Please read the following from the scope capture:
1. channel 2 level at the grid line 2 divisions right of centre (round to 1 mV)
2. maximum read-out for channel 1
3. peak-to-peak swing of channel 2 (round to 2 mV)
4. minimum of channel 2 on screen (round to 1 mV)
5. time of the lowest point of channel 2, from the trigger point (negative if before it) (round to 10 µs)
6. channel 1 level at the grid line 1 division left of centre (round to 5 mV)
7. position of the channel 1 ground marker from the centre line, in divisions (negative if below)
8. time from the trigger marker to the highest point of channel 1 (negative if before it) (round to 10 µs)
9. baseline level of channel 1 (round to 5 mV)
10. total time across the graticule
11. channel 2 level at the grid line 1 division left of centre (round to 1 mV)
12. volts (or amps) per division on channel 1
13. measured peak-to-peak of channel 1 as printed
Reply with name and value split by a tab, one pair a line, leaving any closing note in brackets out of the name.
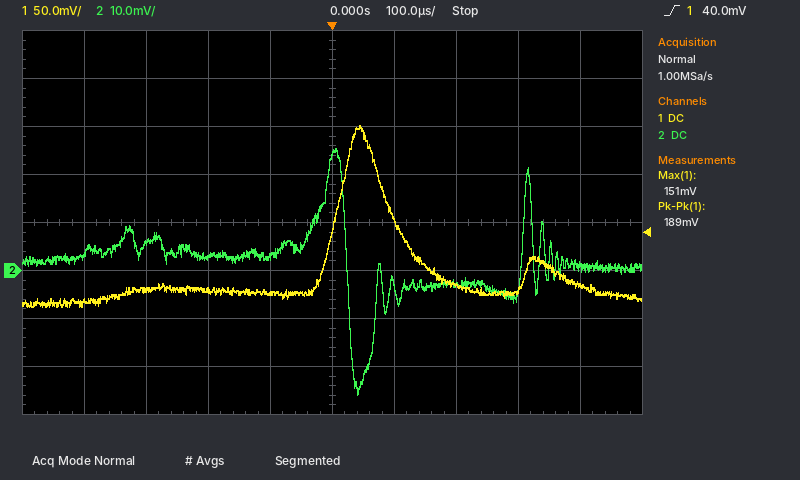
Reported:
channel 2 level at the grid line 2 divisions right of centre	-3 mV
maximum read-out for channel 1	151 mV
peak-to-peak swing of channel 2	52 mV
minimum of channel 2 on screen	-26 mV
time of the lowest point of channel 2, from the trigger point (negative if before it)	+40 µs
channel 1 level at the grid line 1 division left of centre	-25 mV
position of the channel 1 ground marker from the centre line, in divisions	-1.0 div
time from the trigger marker to the highest point of channel 1 (negative if before it)	+40 µs
baseline level of channel 1	-20 mV
total time across the graticule	1 ms
channel 2 level at the grid line 1 division left of centre	3 mV
volts (or amps) per division on channel 1	50 mV
measured peak-to-peak of channel 1 as printed	189 mV
